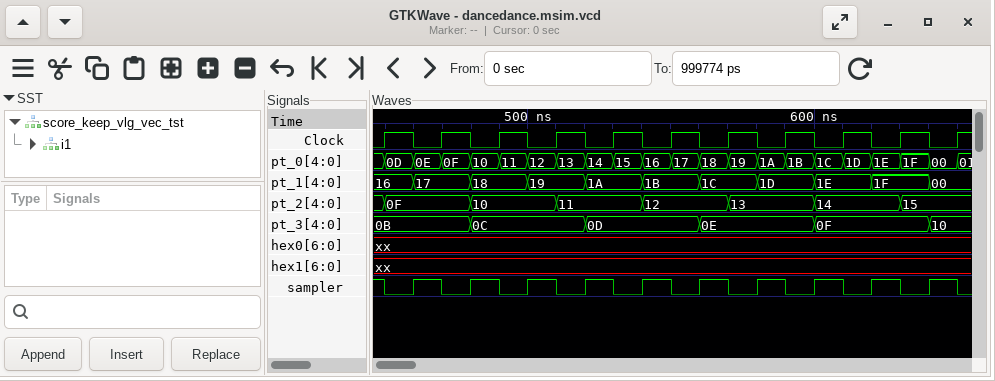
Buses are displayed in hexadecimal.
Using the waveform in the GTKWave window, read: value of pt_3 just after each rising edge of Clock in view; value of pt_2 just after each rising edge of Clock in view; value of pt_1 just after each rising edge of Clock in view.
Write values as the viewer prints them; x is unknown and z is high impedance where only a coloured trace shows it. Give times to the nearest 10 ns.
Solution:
0B, 0B, 0C, 0C, 0D, 0D, 0E, 0E, 0F, 0F, 10
0F, 0F, 10, 11, 11, 12, 13, 13, 14, 15, 15
16, 17, 18, 19, 1A, 1B, 1C, 1D, 1E, 1F, 00
